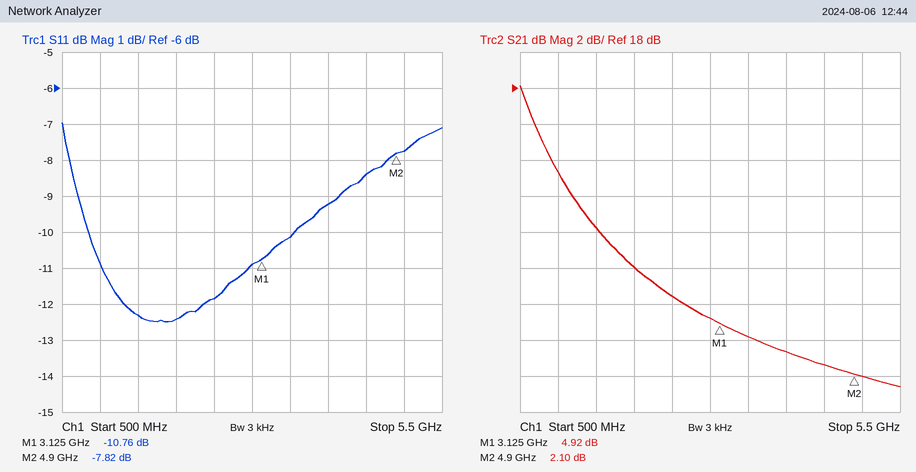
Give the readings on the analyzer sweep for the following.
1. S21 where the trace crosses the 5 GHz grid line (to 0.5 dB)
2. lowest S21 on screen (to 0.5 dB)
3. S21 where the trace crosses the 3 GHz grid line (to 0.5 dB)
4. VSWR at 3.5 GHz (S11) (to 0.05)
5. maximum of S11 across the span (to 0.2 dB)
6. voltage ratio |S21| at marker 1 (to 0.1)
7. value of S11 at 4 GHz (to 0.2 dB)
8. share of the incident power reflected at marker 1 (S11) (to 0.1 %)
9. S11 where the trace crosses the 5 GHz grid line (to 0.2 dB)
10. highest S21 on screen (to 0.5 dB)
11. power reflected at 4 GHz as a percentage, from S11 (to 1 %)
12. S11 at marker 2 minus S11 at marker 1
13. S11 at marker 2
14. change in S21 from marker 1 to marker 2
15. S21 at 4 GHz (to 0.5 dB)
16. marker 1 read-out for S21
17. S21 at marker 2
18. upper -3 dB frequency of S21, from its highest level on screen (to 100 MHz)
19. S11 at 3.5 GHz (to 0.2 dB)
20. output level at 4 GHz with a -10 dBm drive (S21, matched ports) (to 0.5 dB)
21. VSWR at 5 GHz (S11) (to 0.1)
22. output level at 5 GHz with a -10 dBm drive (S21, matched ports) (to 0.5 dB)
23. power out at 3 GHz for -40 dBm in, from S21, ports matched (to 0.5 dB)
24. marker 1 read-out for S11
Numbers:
2.0 dB
1.5 dB
5.0 dB
1.90
-7.0 dB
1.8
-9.2 dB
8.4 %
-7.8 dB
18.0 dB
12 %
2.94 dB
-7.82 dB
-2.82 dB
3.5 dB
4.92 dB
2.10 dB
800 MHz
-10.2 dB
-6.5 dBm
2.4
-8.0 dBm
-35.0 dBm
-10.76 dB
